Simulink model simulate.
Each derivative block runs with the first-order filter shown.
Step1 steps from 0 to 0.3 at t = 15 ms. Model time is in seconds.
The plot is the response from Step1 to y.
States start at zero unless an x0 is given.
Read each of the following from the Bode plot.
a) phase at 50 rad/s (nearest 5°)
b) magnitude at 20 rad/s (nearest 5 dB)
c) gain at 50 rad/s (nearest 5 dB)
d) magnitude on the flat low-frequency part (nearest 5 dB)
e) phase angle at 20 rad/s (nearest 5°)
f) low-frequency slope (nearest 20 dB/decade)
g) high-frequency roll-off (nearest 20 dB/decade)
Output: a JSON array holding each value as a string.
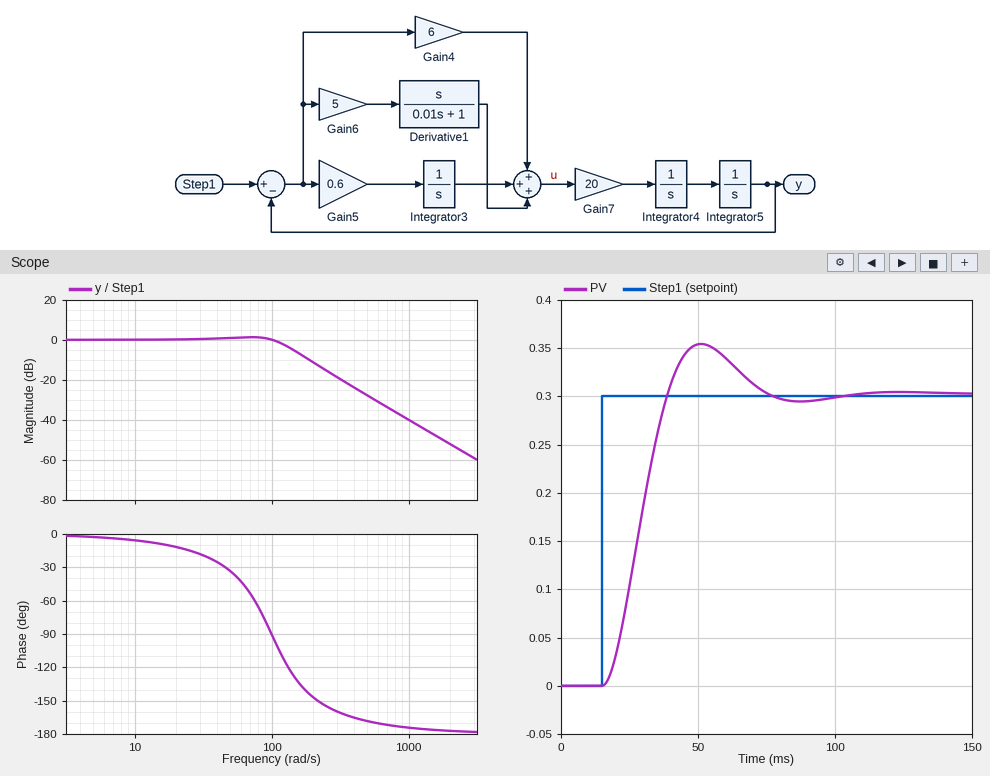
["-35°", "0 dB", "0 dB", "0 dB", "-10°", "0 dB/decade", "-40 dB/decade"]
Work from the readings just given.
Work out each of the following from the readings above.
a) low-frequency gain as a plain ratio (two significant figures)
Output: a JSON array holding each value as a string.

["1.0"]
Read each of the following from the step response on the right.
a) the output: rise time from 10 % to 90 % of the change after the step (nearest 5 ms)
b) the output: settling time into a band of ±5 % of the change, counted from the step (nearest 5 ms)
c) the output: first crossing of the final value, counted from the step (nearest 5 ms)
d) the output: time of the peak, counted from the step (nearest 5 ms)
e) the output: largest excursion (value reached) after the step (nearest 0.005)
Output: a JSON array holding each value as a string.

["15 ms", "55 ms", "25 ms", "35 ms", "0.355"]
